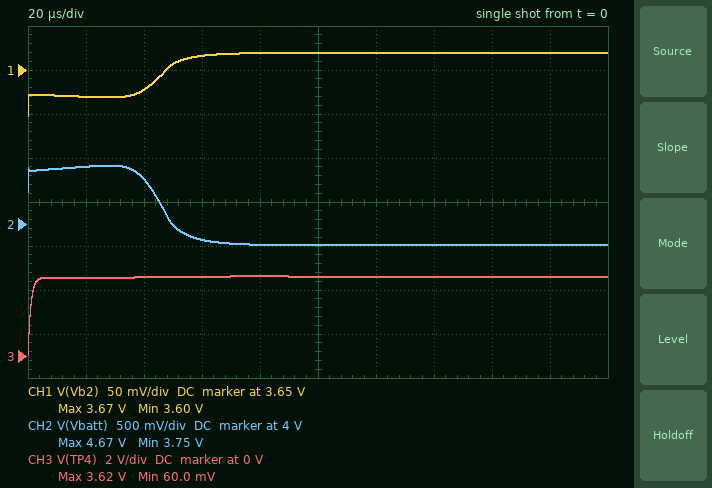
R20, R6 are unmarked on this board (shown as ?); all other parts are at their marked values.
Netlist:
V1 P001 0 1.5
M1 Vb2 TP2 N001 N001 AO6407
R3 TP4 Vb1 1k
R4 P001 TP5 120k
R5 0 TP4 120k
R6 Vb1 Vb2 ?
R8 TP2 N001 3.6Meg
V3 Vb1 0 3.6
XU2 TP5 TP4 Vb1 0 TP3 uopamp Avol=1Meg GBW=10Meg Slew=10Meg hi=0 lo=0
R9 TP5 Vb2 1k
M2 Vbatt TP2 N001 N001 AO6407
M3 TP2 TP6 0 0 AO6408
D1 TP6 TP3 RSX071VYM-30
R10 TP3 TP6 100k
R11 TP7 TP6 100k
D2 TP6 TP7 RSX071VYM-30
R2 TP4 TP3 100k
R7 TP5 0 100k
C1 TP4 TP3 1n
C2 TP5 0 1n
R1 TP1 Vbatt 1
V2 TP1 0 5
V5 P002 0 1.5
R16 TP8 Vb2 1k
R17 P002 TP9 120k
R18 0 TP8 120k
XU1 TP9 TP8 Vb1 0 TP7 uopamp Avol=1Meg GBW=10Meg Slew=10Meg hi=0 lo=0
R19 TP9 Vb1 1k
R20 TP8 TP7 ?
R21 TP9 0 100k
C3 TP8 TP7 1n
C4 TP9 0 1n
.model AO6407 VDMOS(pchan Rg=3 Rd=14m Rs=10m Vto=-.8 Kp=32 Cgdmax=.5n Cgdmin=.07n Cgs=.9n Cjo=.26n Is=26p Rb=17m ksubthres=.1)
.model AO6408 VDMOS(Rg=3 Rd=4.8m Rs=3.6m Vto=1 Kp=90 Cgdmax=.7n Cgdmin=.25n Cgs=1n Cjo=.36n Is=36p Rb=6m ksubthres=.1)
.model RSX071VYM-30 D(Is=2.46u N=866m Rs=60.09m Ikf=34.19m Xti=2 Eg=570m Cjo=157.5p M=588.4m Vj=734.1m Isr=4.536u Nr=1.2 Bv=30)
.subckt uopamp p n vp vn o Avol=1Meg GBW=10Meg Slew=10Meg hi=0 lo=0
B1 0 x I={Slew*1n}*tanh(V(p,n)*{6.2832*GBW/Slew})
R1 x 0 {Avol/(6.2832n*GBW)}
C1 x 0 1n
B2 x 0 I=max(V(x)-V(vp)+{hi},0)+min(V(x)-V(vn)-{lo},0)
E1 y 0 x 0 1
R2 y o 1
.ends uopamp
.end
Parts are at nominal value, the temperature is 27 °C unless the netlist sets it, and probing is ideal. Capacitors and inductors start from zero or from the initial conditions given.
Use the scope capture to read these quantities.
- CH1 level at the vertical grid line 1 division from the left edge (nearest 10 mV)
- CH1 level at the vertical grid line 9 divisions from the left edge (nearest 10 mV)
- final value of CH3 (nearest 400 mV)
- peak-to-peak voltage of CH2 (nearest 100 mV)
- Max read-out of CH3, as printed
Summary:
3.62 V
3.67 V
3.6 V
900 mV
3.62 V
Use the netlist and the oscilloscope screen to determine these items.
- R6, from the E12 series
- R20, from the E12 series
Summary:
0.056 Ω
33 kΩ
